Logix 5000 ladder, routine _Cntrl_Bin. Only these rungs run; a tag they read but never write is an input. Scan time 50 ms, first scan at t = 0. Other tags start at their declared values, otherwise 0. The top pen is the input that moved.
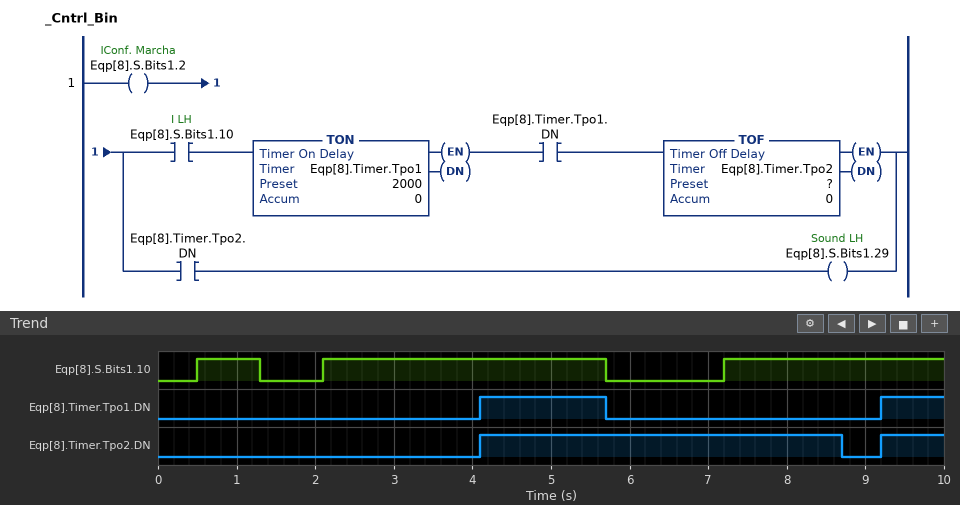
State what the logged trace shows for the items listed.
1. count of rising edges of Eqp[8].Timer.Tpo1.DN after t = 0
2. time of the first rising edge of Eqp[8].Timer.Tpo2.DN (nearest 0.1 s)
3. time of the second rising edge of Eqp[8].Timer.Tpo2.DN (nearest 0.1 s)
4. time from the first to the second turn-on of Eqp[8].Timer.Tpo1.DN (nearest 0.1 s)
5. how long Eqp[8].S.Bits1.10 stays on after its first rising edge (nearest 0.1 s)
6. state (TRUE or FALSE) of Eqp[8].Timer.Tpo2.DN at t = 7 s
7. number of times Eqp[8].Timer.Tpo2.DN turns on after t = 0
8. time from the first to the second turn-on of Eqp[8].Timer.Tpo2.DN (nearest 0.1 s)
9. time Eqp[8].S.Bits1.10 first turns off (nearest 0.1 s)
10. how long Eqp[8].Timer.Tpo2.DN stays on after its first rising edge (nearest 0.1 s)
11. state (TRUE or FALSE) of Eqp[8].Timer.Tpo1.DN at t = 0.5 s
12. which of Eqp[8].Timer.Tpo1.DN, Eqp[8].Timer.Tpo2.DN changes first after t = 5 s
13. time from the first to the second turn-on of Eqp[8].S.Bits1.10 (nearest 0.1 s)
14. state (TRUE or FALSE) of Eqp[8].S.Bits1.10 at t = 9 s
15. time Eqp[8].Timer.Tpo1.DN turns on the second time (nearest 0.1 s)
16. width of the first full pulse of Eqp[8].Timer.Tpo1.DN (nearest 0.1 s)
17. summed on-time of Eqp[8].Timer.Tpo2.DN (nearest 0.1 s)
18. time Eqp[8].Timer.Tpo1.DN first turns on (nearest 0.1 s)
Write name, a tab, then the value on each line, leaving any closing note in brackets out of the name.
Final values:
count of rising edges of Eqp[8].Timer.Tpo1.DN after t = 0	2
time of the first rising edge of Eqp[8].Timer.Tpo2.DN	4.1 s
time of the second rising edge of Eqp[8].Timer.Tpo2.DN	9.2 s
time from the first to the second turn-on of Eqp[8].Timer.Tpo1.DN	5.1 s
how long Eqp[8].S.Bits1.10 stays on after its first rising edge	0.8 s
state (TRUE or FALSE) of Eqp[8].Timer.Tpo2.DN at t = 7 s	TRUE
number of times Eqp[8].Timer.Tpo2.DN turns on after t = 0	2
time from the first to the second turn-on of Eqp[8].Timer.Tpo2.DN	5.1 s
time Eqp[8].S.Bits1.10 first turns off	1.3 s
how long Eqp[8].Timer.Tpo2.DN stays on after its first rising edge	4.6 s
state (TRUE or FALSE) of Eqp[8].Timer.Tpo1.DN at t = 0.5 s	FALSE
which of Eqp[8].Timer.Tpo1.DN, Eqp[8].Timer.Tpo2.DN changes first after t = 5 s	Eqp[8].Timer.Tpo1.DN
time from the first to the second turn-on of Eqp[8].S.Bits1.10	1.6 s
state (TRUE or FALSE) of Eqp[8].S.Bits1.10 at t = 9 s	TRUE
time Eqp[8].Timer.Tpo1.DN turns on the second time	9.2 s
width of the first full pulse of Eqp[8].Timer.Tpo1.DN	1.6 s
summed on-time of Eqp[8].Timer.Tpo2.DN	5.4 s
time Eqp[8].Timer.Tpo1.DN first turns on	4.1 s
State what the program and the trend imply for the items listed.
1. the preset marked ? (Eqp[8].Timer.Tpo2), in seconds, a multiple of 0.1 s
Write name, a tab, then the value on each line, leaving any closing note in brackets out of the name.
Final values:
the preset marked ? (Eqp[8].Timer.Tpo2), in seconds, a multiple of 0.1 s	3.0 s
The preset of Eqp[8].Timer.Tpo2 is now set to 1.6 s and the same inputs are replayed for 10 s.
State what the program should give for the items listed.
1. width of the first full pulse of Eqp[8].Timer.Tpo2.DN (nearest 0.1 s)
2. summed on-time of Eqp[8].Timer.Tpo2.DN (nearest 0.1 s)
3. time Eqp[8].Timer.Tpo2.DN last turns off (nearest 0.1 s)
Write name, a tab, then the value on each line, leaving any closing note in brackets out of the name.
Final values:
width of the first full pulse of Eqp[8].Timer.Tpo2.DN	3.2 s
summed on-time of Eqp[8].Timer.Tpo2.DN	4.0 s
time Eqp[8].Timer.Tpo2.DN last turns off	7.3 s
